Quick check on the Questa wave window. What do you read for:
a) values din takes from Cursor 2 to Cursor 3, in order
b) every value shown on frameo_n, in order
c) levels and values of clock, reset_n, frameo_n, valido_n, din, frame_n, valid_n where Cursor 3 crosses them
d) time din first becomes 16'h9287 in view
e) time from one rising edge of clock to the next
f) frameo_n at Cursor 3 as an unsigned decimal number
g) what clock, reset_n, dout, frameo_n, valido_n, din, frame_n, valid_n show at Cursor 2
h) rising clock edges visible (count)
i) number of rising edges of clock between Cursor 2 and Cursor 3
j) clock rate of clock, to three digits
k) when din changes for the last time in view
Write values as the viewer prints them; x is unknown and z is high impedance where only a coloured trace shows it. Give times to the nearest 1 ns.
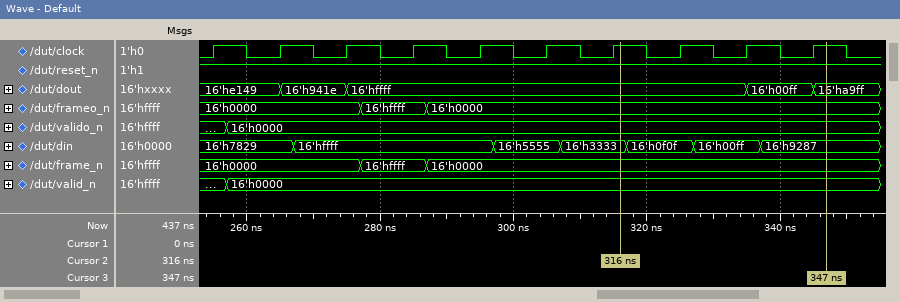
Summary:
16'h3333, 16'h0f0f, 16'h00ff, 16'h9287
16'h0000, 16'hffff, 16'h0000
clock=1, reset_n=1, frameo_n=16'h0000, valido_n=16'h0000, din=16'h9287, frame_n=16'h0000, valid_n=16'h0000
337 ns
10 ns
0
clock=1, reset_n=1, dout=16'hffff, frameo_n=16'h0000, valido_n=16'h0000, din=16'h3333, frame_n=16'h0000, valid_n=16'h0000
10
3
100 MHz
337 ns
